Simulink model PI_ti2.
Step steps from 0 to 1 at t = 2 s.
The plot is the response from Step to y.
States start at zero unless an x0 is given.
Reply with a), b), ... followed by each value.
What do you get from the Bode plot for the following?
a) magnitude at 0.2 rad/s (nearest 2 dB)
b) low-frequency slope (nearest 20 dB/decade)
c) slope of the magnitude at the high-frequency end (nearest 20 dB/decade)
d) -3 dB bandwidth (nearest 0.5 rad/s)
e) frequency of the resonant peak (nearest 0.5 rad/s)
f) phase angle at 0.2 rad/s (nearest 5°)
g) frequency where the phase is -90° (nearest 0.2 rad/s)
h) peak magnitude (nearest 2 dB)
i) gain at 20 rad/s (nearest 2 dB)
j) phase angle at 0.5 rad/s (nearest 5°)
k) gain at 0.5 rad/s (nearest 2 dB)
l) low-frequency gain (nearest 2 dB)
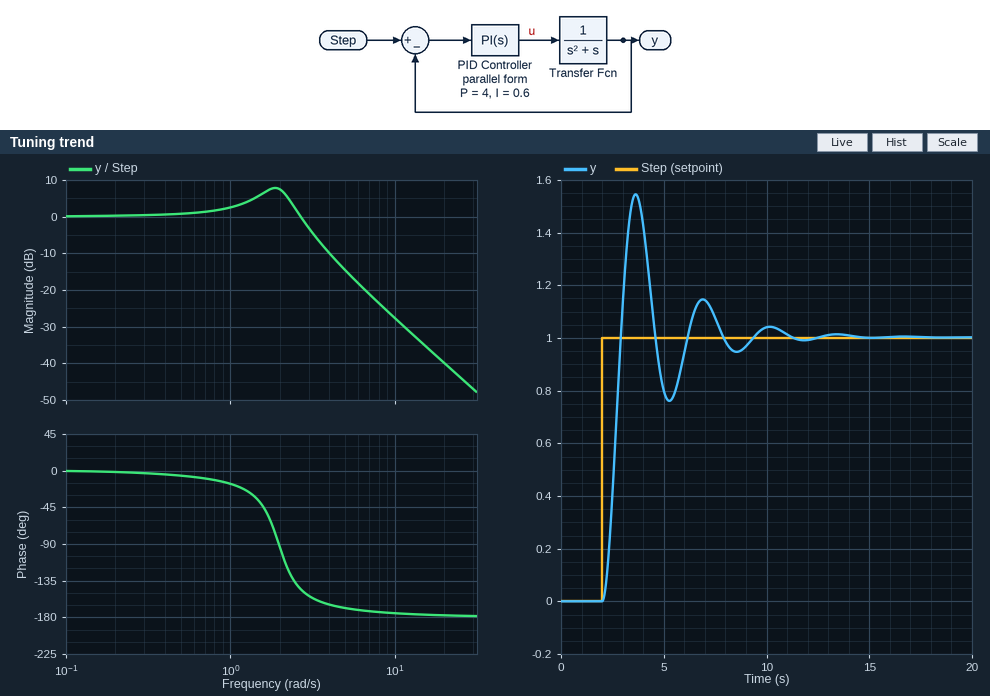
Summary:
a) 0 dB
b) 0 dB/decade
c) -40 dB/decade
d) 3.0 rad/s
e) 2.0 rad/s
f) 0°
g) 2.0 rad/s
h) 8 dB
i) -40 dB
j) -5°
k) 0 dB
l) 0 dB
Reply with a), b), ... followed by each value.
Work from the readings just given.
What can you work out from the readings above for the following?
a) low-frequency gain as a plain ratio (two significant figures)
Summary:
a) 1.0
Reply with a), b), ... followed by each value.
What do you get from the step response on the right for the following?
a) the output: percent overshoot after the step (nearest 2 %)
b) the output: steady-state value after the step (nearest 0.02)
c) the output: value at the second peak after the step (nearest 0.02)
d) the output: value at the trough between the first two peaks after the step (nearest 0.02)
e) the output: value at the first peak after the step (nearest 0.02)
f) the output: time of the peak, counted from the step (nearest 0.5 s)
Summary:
a) 54 %
b) 1.00
c) 1.14
d) 0.76
e) 1.54
f) 1.5 s
